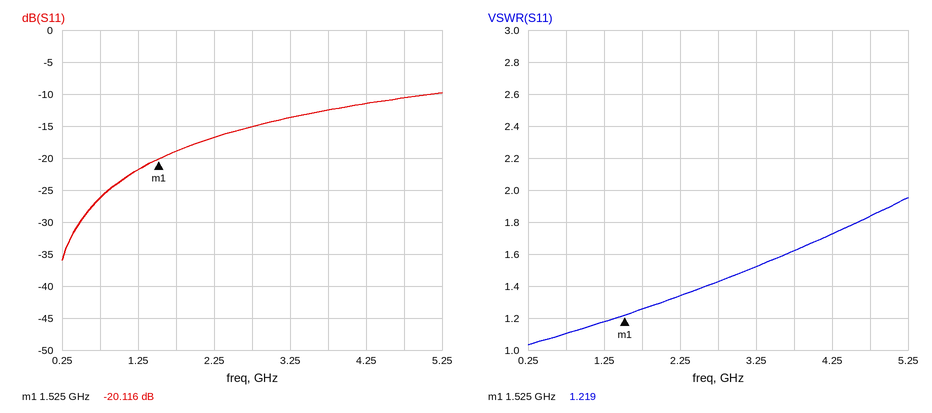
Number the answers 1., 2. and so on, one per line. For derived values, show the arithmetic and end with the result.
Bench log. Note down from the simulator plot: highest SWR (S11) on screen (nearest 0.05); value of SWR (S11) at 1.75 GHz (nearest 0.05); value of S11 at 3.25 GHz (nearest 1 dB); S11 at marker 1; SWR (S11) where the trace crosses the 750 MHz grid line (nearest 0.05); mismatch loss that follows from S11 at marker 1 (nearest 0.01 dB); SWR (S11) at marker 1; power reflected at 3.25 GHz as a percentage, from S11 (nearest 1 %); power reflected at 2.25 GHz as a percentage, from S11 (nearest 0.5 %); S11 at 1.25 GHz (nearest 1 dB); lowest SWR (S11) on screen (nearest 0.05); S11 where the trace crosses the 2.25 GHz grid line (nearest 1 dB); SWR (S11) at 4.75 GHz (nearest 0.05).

1. 1.95
2. 1.25
3. -14 dB
4. -20.116 dB
5. 1.10
6. −10 log10(1 − 10^(-20.116/10)) ≈ 0.04 dB
7. 1.219
8. 10^(-14/10) ≈ 4 %
9. 10^(-17/10) ≈ 2.0 %
10. -22 dB
11. 1.05
12. -17 dB
13. 1.85
